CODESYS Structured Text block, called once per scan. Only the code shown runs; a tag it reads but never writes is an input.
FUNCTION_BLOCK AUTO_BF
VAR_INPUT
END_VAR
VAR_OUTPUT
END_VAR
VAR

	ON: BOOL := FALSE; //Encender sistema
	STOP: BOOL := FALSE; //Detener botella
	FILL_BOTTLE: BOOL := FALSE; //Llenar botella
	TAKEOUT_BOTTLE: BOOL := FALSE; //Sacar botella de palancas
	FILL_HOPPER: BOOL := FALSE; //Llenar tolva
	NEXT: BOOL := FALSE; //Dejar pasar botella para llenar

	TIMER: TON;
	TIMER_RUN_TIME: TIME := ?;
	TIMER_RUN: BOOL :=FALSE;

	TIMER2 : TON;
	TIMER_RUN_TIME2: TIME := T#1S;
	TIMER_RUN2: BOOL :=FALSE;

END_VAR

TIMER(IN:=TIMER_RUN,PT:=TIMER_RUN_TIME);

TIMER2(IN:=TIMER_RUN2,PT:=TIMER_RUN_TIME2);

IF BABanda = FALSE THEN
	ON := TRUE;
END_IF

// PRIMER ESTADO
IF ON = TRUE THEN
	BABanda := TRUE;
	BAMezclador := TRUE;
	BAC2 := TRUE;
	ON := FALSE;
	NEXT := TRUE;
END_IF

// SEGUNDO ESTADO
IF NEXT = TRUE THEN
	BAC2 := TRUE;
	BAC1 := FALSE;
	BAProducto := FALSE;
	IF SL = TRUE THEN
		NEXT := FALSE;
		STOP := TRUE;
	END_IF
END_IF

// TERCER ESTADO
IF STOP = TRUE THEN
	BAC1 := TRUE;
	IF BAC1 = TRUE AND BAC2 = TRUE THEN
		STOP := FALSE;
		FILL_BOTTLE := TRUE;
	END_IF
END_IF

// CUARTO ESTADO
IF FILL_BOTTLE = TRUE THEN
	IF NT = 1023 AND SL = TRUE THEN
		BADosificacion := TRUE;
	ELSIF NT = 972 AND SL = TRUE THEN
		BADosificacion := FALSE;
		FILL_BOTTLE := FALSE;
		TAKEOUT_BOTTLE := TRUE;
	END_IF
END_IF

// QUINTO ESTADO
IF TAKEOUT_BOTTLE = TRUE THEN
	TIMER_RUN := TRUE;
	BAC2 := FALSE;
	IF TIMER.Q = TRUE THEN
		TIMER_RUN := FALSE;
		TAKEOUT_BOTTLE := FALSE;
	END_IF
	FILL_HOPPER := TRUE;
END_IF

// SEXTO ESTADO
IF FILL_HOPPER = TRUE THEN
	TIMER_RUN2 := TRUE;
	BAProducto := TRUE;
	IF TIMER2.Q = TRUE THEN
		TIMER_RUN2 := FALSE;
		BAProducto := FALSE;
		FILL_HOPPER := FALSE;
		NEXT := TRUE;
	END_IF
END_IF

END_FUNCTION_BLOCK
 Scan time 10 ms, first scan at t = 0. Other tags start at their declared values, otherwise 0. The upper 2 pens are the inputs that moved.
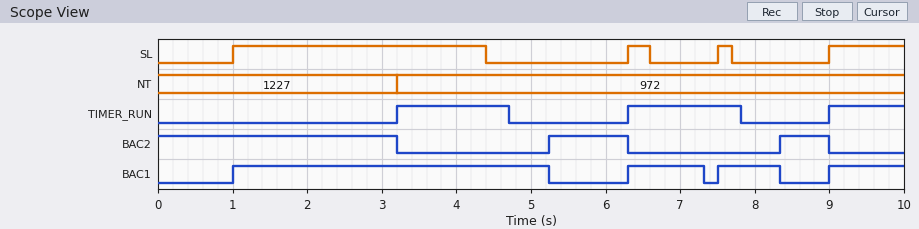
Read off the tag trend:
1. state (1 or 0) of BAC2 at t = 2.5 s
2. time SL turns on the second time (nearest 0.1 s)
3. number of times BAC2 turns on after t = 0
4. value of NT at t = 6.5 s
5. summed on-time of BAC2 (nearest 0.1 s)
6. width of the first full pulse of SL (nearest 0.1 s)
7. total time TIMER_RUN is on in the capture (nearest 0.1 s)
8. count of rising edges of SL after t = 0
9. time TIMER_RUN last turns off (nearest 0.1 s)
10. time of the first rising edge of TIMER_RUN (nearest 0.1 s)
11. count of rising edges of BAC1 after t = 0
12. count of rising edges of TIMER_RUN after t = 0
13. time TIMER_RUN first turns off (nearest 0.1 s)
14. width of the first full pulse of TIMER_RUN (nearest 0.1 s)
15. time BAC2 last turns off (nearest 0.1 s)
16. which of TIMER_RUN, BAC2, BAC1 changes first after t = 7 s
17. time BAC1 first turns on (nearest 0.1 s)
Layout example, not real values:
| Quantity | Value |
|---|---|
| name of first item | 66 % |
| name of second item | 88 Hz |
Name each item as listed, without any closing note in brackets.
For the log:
| Quantity | Value |
|---|---|
| state (1 or 0) of BAC2 at t = 2.5 s | 1 |
| time SL turns on the second time | 6.3 s |
| number of times BAC2 turns on after t = 0 | 2 |
| value of NT at t = 6.5 s | 972 |
| summed on-time of BAC2 | 4.9 s |
| width of the first full pulse of SL | 3.4 s |
| total time TIMER_RUN is on in the capture | 4.0 s |
| count of rising edges of SL after t = 0 | 4 |
| time TIMER_RUN last turns off | 7.8 s |
| time of the first rising edge of TIMER_RUN | 3.2 s |
| count of rising edges of BAC1 after t = 0 | 4 |
| count of rising edges of TIMER_RUN after t = 0 | 3 |
| time TIMER_RUN first turns off | 4.7 s |
| width of the first full pulse of TIMER_RUN | 1.5 s |
| time BAC2 last turns off | 9.0 s |
| which of TIMER_RUN, BAC2, BAC1 changes first after t = 7 s | BAC1 |
| time BAC1 first turns on | 1.0 s |
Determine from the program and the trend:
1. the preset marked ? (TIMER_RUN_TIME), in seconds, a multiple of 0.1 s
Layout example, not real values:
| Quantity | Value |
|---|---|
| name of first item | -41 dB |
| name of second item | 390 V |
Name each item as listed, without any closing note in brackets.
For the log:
| Quantity | Value |
|---|---|
| the preset marked ? (TIMER_RUN_TIME), in seconds, a multiple of 0.1 s | 1.5 s |
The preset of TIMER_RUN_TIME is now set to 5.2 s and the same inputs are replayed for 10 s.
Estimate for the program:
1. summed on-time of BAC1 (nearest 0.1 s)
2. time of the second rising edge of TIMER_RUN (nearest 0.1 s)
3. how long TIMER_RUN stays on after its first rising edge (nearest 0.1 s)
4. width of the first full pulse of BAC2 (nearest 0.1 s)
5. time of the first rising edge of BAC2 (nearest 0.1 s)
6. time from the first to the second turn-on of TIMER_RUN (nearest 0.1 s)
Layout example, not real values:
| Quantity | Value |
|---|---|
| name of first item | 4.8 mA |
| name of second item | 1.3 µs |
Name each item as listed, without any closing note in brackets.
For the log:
| Quantity | Value |
|---|---|
| summed on-time of BAC1 | 7.0 s |
| time of the second rising edge of TIMER_RUN | 9.0 s |
| how long TIMER_RUN stays on after its first rising edge | 5.2 s |
| width of the first full pulse of BAC2 | 0.6 s |
| time of the first rising edge of BAC2 | 8.4 s |
| time from the first to the second turn-on of TIMER_RUN | 5.8 s |
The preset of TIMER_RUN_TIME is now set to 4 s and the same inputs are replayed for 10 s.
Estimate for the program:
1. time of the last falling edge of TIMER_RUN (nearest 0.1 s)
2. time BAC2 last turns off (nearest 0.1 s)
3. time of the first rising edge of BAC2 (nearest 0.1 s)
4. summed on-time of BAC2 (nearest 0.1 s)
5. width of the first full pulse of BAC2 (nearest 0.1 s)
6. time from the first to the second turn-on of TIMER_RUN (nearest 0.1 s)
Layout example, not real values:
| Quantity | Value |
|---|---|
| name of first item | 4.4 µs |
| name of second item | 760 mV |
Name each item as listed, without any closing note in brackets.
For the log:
| Quantity | Value |
|---|---|
| time of the last falling edge of TIMER_RUN | 7.2 s |
| time BAC2 last turns off | 7.5 s |
| time of the first rising edge of BAC2 | 7.3 s |
| summed on-time of BAC2 | 3.4 s |
| width of the first full pulse of BAC2 | 0.2 s |
| time from the first to the second turn-on of TIMER_RUN | 4.3 s |
